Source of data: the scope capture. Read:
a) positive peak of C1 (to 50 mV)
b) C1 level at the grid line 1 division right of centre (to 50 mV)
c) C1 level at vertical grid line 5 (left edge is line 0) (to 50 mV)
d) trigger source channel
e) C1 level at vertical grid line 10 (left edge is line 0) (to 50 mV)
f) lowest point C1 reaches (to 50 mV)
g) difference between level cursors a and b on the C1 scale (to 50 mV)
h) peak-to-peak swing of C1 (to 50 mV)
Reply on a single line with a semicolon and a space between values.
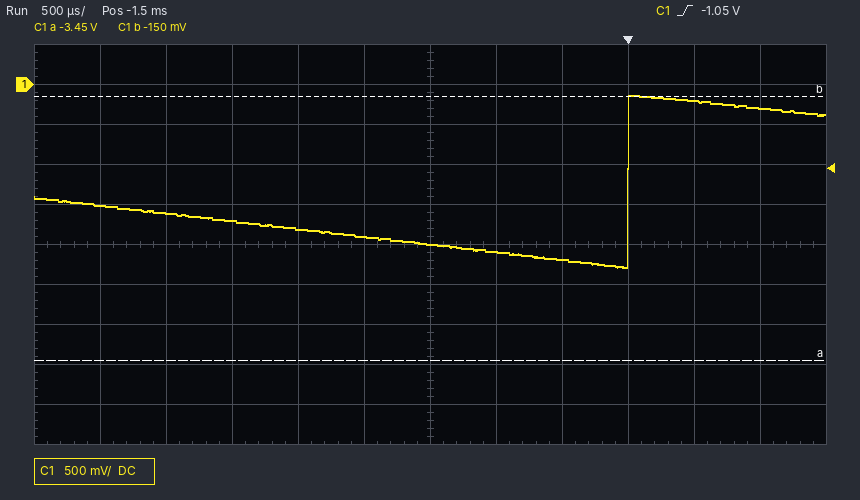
-150 mV; -2.10 V; -1.90 V; C1; -200 mV; -2.30 V; 3.30 V; 2.15 V
